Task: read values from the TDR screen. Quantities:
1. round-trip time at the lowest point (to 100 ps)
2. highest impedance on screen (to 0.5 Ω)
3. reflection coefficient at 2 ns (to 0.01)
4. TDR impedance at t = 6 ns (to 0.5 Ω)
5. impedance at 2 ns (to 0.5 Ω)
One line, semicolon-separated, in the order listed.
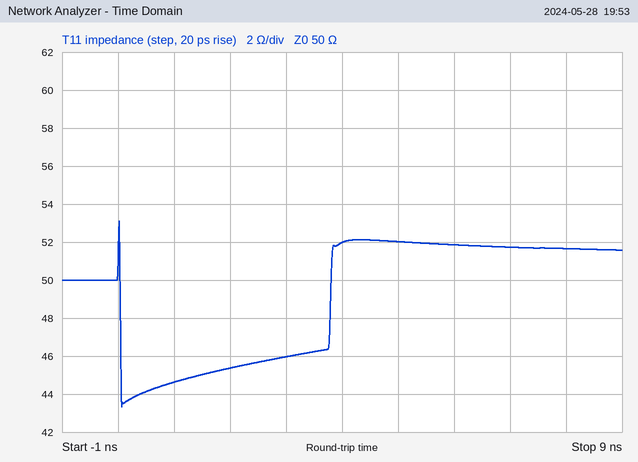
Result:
100 ps; 53.0 Ω; -0.05; 52.0 Ω; 45.5 Ω
